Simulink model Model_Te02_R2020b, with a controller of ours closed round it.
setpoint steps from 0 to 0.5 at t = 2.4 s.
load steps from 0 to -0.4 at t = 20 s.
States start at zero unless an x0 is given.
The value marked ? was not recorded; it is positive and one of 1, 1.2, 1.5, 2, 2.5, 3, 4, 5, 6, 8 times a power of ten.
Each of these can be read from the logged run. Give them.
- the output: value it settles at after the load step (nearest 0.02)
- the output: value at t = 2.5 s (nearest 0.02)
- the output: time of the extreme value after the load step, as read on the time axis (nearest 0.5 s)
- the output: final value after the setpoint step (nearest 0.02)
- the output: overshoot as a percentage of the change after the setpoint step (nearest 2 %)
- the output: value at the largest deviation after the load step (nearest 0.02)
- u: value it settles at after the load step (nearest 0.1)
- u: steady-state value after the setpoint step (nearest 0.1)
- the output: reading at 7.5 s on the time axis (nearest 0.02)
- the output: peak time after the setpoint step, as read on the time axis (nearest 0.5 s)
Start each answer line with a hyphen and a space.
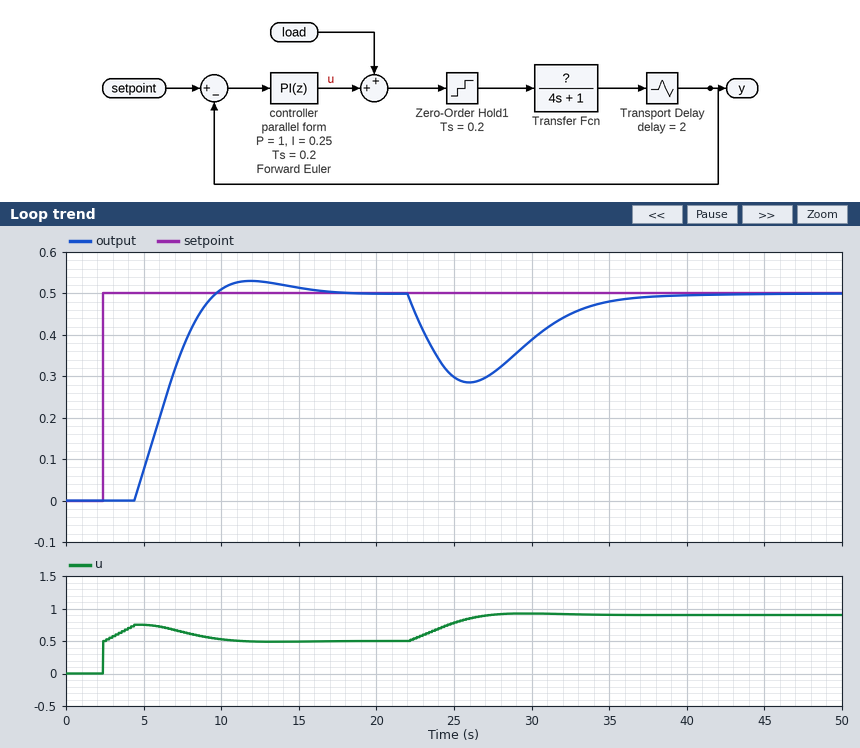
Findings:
- 0.50
- 0.00
- 26.0 s
- 0.50
- 6 %
- 0.28
- 0.9
- 0.5
- 0.36
- 12.0 s
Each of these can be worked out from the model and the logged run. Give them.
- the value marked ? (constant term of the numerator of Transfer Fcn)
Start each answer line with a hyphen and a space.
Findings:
- 1
